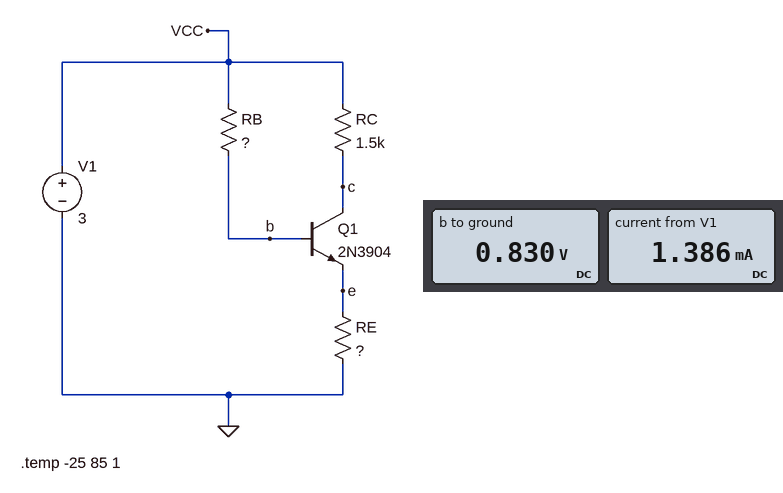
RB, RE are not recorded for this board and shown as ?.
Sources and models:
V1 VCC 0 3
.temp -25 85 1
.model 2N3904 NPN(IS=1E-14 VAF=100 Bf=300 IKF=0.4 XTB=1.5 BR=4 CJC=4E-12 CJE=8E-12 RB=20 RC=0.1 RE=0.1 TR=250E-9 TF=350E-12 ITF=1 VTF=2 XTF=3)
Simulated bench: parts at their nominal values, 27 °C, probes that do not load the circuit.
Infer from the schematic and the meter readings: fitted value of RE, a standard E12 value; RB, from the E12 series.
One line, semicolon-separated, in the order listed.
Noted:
120 Ω; 470 kΩ
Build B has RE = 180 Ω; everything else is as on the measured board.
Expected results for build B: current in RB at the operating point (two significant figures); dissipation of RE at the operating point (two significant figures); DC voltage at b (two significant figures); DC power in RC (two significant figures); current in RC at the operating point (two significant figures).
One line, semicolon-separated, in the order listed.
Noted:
4.5 µA; 320 µW; 900 mV; 2.7 mW; 1.3 mA
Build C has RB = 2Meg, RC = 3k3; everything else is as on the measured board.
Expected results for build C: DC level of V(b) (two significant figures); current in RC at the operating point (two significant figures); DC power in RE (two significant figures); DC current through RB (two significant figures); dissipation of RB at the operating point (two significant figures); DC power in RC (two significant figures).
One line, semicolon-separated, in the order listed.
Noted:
670 mV; 350 µA; 15 µW; 1.2 µA; 2.7 µW; 410 µW
